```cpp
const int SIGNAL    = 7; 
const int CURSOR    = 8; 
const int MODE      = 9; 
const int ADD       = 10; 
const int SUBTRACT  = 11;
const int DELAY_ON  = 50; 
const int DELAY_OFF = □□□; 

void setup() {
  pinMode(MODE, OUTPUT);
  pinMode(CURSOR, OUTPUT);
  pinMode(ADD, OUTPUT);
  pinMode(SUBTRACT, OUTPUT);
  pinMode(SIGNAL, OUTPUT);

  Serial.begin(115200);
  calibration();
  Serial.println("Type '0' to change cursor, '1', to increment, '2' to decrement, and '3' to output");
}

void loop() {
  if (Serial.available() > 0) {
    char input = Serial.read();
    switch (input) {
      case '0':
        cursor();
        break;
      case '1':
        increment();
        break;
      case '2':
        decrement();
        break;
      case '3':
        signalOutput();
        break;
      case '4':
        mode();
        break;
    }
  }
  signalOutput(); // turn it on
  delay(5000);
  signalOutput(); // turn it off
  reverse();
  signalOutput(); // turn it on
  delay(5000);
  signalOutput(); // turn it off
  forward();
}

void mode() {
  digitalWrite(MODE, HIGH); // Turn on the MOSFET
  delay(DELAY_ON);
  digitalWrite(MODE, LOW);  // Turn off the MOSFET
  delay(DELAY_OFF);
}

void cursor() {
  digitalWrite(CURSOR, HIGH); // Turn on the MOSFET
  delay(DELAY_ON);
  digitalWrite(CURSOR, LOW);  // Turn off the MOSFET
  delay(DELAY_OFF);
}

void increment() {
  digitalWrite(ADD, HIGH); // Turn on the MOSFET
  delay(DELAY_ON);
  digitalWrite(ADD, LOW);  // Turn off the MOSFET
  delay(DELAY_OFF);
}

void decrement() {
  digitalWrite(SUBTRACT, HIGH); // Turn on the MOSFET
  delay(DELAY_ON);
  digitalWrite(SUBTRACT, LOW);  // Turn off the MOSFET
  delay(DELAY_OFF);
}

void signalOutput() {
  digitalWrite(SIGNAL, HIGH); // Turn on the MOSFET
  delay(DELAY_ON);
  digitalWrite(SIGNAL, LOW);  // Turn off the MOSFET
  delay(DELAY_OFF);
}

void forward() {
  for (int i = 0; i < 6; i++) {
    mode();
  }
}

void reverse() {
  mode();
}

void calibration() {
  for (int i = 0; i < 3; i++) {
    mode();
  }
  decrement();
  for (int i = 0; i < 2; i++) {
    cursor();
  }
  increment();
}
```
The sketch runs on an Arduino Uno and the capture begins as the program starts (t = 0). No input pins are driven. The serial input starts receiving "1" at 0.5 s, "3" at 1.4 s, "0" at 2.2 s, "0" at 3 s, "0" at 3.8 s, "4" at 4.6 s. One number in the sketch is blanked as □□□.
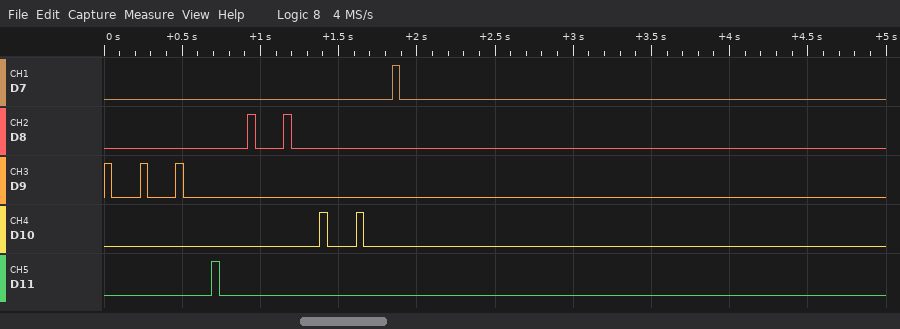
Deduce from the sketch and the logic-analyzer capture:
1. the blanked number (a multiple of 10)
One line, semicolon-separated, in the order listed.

180
